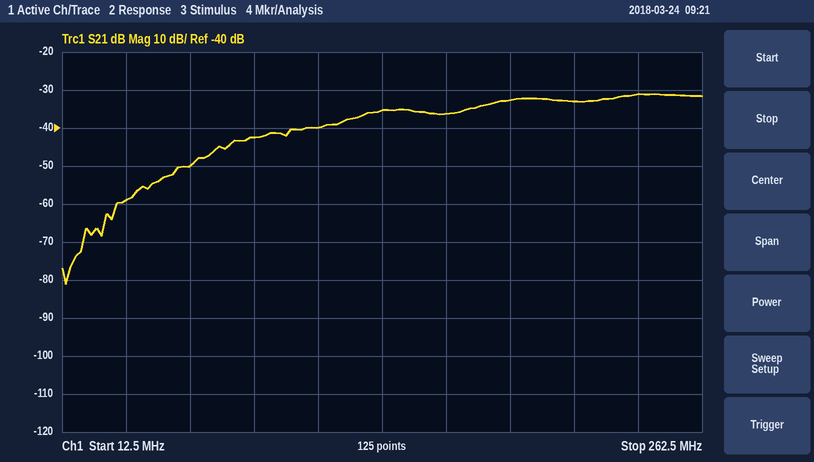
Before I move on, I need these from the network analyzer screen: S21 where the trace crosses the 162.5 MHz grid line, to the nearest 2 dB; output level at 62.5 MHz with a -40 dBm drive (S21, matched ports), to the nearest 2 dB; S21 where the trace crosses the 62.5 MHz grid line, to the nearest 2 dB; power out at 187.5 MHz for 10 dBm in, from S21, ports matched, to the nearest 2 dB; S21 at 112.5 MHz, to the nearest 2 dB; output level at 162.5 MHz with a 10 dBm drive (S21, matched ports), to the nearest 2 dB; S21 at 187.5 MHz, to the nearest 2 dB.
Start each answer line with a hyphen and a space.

- -36 dB
- -90 dBm
- -50 dB
- -22 dBm
- -40 dB
- -26 dBm
- -32 dB
